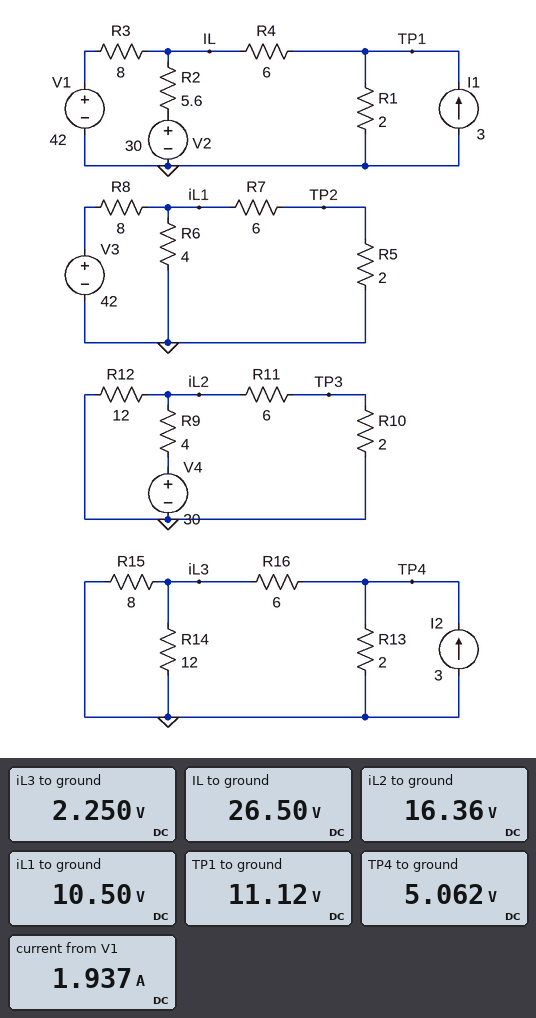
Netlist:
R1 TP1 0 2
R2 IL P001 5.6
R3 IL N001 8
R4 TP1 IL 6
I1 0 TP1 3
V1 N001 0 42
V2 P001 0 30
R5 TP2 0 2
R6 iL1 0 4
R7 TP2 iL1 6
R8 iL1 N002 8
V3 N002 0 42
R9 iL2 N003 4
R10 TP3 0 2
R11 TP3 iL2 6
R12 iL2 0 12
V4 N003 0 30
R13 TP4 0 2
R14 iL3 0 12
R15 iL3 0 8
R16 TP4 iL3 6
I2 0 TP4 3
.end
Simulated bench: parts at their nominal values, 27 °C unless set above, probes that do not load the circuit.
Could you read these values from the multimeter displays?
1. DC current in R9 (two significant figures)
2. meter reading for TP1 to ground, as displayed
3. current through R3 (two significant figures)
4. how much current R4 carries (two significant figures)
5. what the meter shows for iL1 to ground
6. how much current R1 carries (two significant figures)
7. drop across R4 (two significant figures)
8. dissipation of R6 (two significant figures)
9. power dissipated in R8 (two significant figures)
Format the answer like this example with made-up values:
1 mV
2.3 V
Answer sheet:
3.4 A
11.12 V
1.9 A
2.6 A
10.50 V
5.6 A
15 V
28 W
120 W
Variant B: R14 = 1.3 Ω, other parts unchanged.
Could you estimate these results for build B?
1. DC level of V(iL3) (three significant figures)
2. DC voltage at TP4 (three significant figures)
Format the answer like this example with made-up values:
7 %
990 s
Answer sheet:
736 mV
4.68 V
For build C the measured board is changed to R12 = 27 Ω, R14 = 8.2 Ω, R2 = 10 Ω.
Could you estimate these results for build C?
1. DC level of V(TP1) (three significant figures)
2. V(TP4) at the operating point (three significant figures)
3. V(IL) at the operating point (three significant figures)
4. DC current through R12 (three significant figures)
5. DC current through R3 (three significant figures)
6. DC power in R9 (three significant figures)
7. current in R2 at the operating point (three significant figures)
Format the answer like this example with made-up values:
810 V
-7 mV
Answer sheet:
10.9 V
5.00 V
25.7 V
674 mA
2.04 A
34.8 W
429 mA
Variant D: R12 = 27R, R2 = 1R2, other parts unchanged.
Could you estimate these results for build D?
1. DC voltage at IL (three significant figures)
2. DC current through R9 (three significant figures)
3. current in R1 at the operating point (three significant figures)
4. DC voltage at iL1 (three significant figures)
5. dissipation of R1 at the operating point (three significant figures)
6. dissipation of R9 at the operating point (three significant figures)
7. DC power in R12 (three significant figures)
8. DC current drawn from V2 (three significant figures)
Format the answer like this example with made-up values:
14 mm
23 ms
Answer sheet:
28.6 V
2.95 A
5.83 A
10.5 V
67.9 W
34.8 W
12.3 W
1.15 A
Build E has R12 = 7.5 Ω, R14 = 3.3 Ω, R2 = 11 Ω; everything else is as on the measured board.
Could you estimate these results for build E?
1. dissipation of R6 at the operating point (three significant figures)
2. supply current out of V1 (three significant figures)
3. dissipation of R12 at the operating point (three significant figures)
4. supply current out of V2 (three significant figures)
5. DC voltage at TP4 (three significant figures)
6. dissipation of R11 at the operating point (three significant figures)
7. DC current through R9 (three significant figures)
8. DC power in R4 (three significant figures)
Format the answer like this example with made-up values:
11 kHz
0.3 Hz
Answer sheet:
27.6 W
2.05 A
29.0 W
400 mA
4.84 V
20.4 W
3.81 A
36.0 W
